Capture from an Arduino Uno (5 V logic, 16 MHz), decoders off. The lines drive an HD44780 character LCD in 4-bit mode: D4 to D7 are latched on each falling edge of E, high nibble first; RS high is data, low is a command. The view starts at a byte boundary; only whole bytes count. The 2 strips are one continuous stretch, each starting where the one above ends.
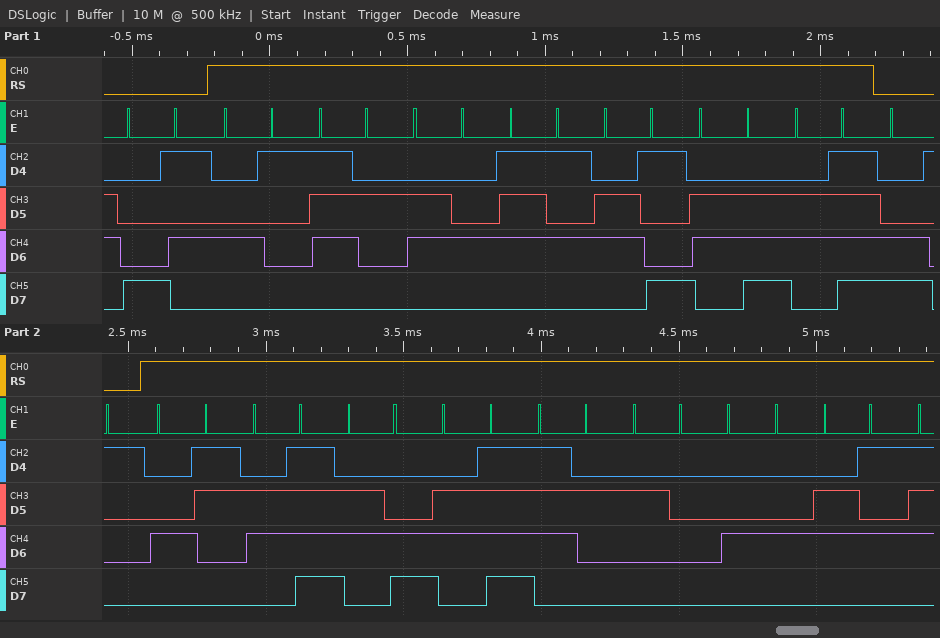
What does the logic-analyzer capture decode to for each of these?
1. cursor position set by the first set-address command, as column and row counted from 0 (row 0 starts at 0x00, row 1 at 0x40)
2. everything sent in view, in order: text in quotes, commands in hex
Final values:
column 5, row 0
0x85 "Arduino" 0xC1 "Color De"
